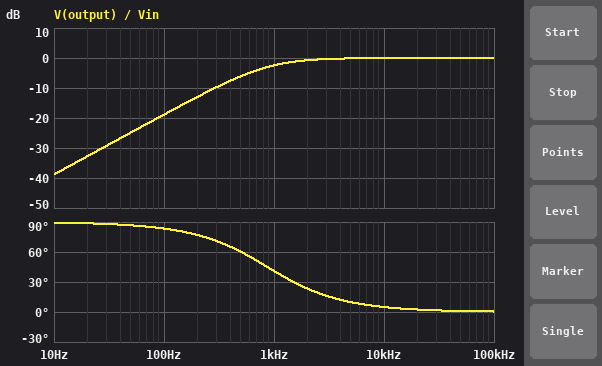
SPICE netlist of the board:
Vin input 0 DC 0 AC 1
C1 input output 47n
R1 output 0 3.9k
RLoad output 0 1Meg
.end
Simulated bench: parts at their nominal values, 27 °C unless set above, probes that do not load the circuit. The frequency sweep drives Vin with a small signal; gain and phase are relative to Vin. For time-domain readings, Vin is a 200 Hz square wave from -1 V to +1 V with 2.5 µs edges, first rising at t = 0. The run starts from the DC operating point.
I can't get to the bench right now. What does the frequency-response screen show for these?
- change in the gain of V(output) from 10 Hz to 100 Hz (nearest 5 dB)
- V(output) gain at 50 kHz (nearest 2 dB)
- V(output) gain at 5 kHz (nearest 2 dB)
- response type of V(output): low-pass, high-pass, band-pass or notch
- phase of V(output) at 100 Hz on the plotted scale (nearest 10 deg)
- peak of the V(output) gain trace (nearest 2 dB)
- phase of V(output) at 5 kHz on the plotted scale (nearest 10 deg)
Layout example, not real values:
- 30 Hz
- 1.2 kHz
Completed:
- 20 dB
- 0 dB
- 0 dB
- high-pass
- 80 deg
- 0 dB
- 10 deg
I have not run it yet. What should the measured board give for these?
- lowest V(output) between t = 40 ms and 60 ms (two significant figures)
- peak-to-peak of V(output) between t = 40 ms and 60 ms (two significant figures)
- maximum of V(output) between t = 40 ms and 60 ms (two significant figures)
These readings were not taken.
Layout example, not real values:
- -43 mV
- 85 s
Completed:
- -2.0 V
- 4.0 V
- 2.0 V
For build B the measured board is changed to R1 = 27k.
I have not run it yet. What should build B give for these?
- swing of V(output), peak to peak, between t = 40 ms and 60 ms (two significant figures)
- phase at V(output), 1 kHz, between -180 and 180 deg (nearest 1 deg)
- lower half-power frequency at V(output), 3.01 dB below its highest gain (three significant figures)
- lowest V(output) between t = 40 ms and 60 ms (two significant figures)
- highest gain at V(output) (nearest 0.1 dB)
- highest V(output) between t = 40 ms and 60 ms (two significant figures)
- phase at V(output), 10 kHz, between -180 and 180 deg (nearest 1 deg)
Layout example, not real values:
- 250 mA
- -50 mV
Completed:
- 3.5 V
- 7 deg
- 129 Hz
- -1.8 V
- 0 dB
- 1.8 V
- 1 deg
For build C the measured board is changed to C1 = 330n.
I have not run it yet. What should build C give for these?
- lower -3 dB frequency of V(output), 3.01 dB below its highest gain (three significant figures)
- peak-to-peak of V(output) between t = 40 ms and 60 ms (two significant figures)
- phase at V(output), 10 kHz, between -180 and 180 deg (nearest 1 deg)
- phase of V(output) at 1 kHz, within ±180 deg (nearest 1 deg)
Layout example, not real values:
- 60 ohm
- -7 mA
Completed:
- 124 Hz
- 3.5 V
- 1 deg
- 7 deg
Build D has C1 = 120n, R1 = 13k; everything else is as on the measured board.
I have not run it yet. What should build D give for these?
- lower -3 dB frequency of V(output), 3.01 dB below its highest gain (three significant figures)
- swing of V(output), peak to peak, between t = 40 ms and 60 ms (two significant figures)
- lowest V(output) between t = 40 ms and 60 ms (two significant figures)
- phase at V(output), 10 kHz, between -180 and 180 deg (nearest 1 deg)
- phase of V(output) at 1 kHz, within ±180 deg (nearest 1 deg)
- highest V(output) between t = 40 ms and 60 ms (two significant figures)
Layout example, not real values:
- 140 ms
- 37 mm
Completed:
- 103 Hz
- 3.3 V
- -1.7 V
- 1 deg
- 6 deg
- 1.7 V
